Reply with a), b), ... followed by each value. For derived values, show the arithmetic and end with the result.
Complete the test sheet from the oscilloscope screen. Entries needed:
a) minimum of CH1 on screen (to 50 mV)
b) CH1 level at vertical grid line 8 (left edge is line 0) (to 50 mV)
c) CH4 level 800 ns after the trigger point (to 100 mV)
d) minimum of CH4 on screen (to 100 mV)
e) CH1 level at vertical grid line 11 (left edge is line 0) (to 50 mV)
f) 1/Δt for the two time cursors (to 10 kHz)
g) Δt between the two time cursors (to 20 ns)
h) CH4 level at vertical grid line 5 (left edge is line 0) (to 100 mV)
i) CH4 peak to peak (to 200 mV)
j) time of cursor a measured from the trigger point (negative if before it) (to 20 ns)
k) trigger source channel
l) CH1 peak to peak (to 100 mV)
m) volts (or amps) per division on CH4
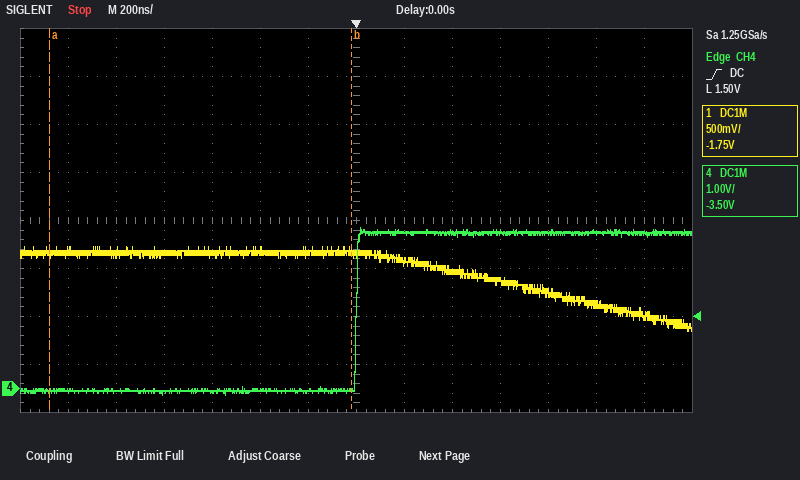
a) 600 mV
b) 1.30 V
c) 3.2 V
d) -100 mV
e) 1.00 V
f) 1 / 1.26 µs ≈ 790 kHz
g) 1.26 µs
h) 0.0 V
i) 3.4 V
j) -1.28 µs
k) CH4
l) 900 mV
m) 1 V
